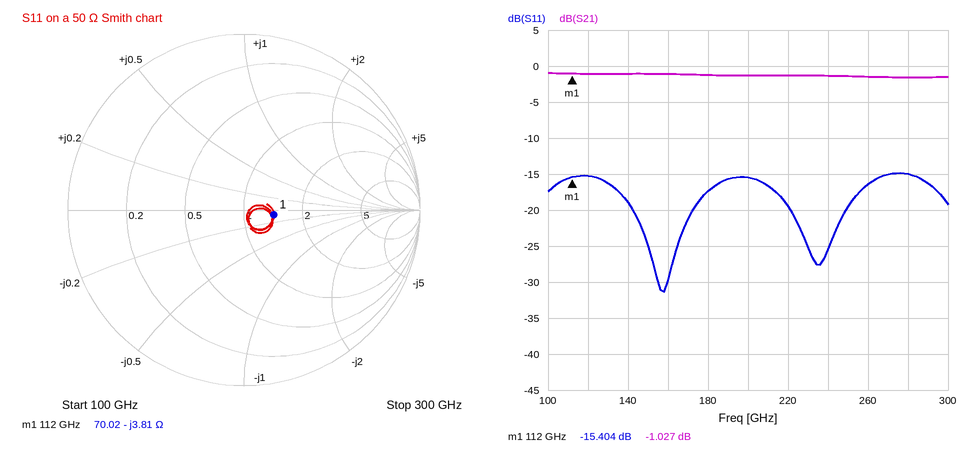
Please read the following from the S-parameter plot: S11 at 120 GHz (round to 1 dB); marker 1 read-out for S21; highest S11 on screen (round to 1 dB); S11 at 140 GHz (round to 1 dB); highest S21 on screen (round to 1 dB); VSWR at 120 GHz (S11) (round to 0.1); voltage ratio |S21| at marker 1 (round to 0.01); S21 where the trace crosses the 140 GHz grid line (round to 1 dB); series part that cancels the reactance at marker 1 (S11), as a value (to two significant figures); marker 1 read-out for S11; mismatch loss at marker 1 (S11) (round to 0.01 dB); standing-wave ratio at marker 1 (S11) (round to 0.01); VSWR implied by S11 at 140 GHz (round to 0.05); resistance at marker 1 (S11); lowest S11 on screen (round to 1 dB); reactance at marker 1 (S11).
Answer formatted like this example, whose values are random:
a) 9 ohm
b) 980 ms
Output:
a) -15 dB
b) -1.027 dB
c) -15 dB
d) -19 dB
e) -1 dB
f) 1.4
g) 0.89
h) -1 dB
i) 5.4 pH
j) -15.404 dB
k) 0.13 dB
l) 1.41
m) 1.25
n) 70.02 Ω
o) -31 dB
p) -3.81 Ω
